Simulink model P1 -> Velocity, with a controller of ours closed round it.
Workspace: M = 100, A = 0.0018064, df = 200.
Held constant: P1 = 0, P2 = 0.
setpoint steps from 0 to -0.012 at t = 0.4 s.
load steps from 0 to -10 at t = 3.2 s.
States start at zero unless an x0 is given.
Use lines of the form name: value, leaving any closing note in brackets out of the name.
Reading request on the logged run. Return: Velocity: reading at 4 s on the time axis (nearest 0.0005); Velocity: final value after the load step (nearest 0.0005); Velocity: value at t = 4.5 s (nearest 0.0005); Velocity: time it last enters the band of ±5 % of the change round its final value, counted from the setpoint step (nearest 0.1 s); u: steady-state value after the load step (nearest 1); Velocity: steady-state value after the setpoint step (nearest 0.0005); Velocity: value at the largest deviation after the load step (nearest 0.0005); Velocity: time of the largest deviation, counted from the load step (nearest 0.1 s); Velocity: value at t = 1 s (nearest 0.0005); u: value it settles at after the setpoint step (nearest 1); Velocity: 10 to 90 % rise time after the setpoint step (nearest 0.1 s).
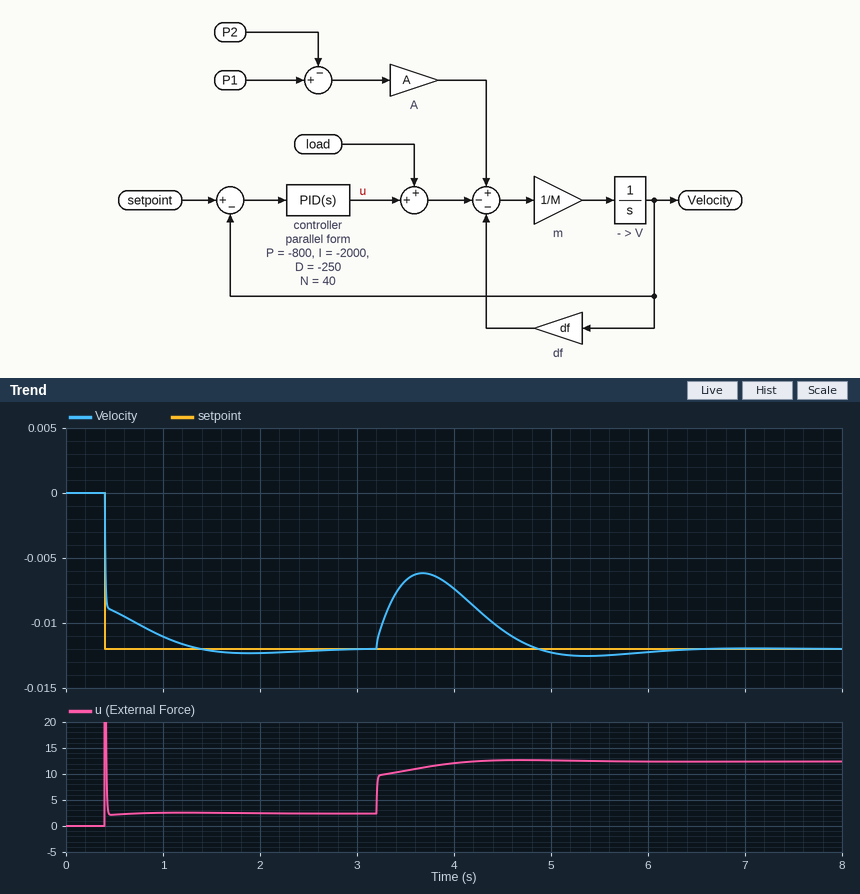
Velocity: reading at 4 s on the time axis: -0.0075
Velocity: final value after the load step: -0.0120
Velocity: value at t = 4.5 s: -0.0105
Velocity: time it last enters the band of ±5 % of the change round its final value, counted from the setpoint step: 0.7 s
u: steady-state value after the load step: 12
Velocity: steady-state value after the setpoint step: -0.0120
Velocity: value at the largest deviation after the load step: -0.0060
Velocity: time of the largest deviation, counted from the load step: 0.5 s
Velocity: value at t = 1 s: -0.0110
u: value it settles at after the setpoint step: 2
Velocity: 10 to 90 % rise time after the setpoint step: 0.5 s
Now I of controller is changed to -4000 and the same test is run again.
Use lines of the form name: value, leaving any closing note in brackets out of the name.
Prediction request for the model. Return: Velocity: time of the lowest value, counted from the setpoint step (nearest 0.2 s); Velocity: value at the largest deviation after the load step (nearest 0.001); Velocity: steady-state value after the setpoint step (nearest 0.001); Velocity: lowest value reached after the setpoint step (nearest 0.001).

Velocity: time of the lowest value, counted from the setpoint step: 1.0 s
Velocity: value at the largest deviation after the load step: -0.007
Velocity: steady-state value after the setpoint step: -0.012
Velocity: lowest value reached after the setpoint step: -0.013
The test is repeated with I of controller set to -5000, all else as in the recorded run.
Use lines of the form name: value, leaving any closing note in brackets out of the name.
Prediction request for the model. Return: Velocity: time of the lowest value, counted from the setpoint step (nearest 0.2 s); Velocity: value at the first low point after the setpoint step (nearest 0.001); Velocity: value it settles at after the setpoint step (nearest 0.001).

Velocity: time of the lowest value, counted from the setpoint step: 0.8 s
Velocity: value at the first low point after the setpoint step: -0.013
Velocity: value it settles at after the setpoint step: -0.012
